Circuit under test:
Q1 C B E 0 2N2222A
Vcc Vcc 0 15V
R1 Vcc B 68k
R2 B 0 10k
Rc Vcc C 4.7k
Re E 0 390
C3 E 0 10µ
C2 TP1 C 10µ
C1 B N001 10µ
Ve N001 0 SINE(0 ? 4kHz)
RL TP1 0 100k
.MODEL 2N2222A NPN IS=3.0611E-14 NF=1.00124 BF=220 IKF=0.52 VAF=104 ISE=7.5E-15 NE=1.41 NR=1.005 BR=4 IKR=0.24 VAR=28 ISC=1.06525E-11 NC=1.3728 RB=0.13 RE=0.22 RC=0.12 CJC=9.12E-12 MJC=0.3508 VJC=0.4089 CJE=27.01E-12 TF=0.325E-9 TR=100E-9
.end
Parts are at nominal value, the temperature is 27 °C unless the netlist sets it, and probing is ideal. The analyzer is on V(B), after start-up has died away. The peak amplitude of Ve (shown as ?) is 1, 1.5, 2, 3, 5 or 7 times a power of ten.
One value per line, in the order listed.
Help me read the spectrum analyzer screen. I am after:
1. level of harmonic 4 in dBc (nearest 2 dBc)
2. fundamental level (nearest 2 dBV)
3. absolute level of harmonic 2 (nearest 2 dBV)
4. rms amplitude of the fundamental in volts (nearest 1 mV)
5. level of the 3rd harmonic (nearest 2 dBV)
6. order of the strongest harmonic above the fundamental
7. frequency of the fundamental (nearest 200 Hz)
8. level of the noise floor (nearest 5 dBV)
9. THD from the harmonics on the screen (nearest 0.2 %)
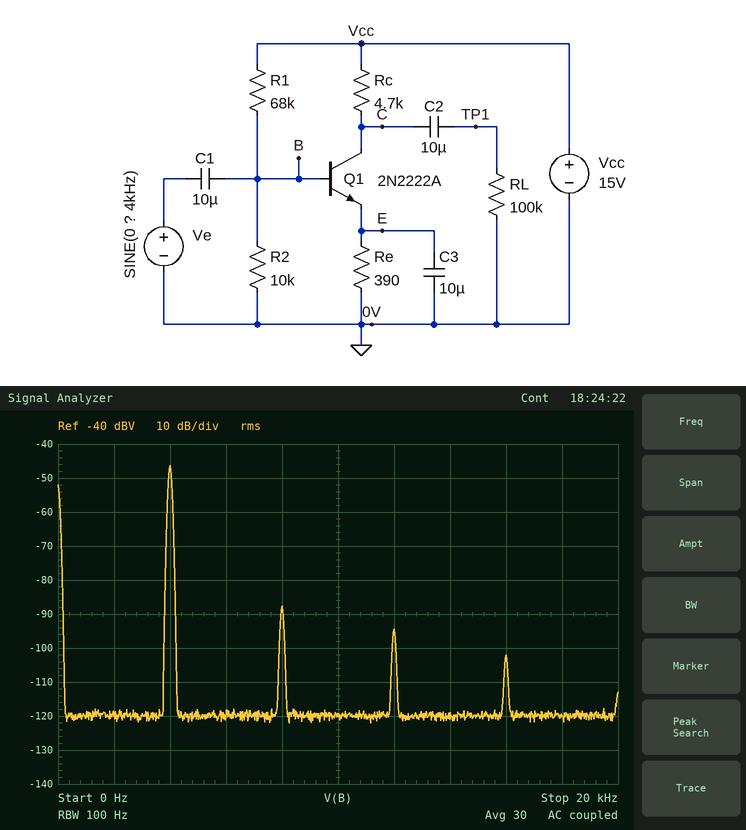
-56 dBc
-46 dBV
-88 dBV
5 mV
-94 dBV
2
4.0 kHz
-120 dBV
1.0 %
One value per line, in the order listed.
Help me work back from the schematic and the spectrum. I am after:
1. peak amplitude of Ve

7 mV
